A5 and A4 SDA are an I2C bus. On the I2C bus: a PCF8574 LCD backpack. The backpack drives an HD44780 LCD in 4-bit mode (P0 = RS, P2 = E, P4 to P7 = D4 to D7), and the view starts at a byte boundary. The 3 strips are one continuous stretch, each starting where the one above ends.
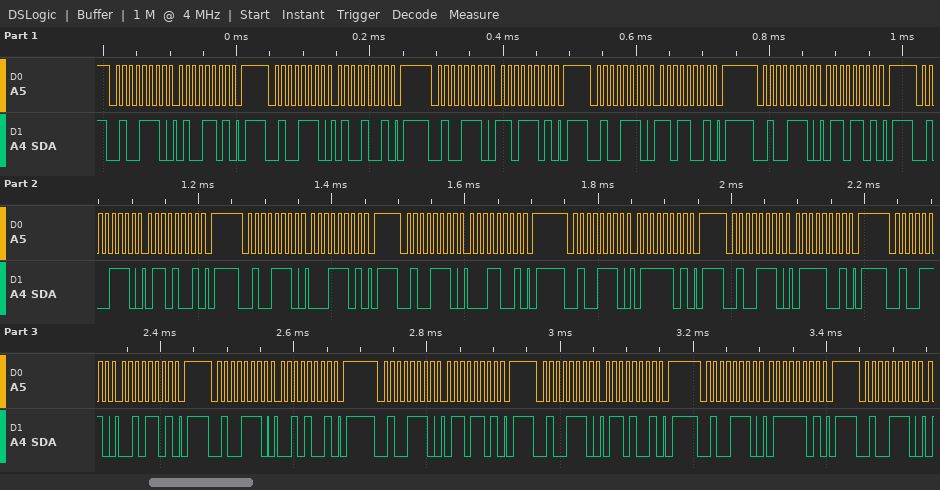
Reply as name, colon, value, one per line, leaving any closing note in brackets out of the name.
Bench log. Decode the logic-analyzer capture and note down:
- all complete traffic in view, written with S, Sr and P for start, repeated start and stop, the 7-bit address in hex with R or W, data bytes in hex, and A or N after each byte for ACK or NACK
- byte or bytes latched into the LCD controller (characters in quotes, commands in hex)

all complete traffic in view, written with S, Sr and P for start, repeated start and stop, the 7-bit address in hex with R or W, data bytes in hex, and A or N after each byte for ACK or NACK: S 27W A 4D A P S 27W A 49 A P S 27W A DD A P S 27W A D9 A P S 27W A 6D A P S 27W A 69 A P S 27W A 1D A P S 27W A 19 A P S 27W A 7D A P S 27W A 79 A P S 27W A 2D A P S 27W A 29 A P S 27W A 6D A P S 27W A 69 A P S 27W A 7D A P S 27W A
byte or bytes latched into the LCD controller: 'M' 'a' 'r'
